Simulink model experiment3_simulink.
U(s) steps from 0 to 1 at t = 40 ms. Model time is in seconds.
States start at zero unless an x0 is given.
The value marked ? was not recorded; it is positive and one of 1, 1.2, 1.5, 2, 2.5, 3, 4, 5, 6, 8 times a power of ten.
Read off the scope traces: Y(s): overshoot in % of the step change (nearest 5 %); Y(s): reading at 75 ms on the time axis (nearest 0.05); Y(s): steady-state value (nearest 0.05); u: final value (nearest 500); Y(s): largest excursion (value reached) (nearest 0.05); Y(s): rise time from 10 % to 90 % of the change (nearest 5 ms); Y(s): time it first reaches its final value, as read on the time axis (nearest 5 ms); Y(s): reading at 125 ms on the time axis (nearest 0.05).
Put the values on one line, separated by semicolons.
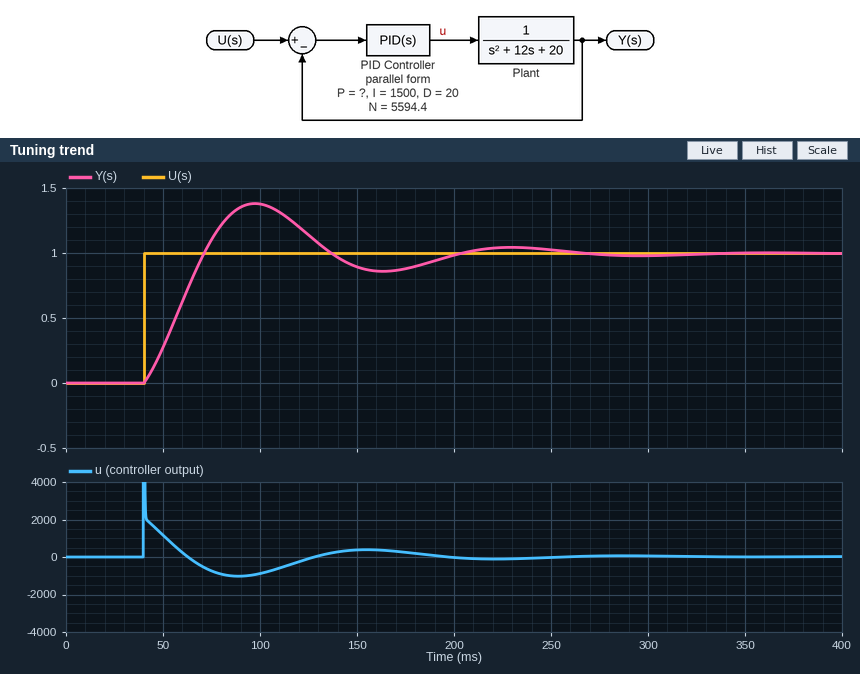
40 %; 1.10; 1.00; 0; 1.40; 25 ms; 70 ms; 1.15
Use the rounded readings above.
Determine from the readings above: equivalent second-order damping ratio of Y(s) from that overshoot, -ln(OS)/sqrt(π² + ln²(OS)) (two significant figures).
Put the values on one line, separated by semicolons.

0.28
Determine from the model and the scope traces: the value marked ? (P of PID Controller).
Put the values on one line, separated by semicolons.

2500
